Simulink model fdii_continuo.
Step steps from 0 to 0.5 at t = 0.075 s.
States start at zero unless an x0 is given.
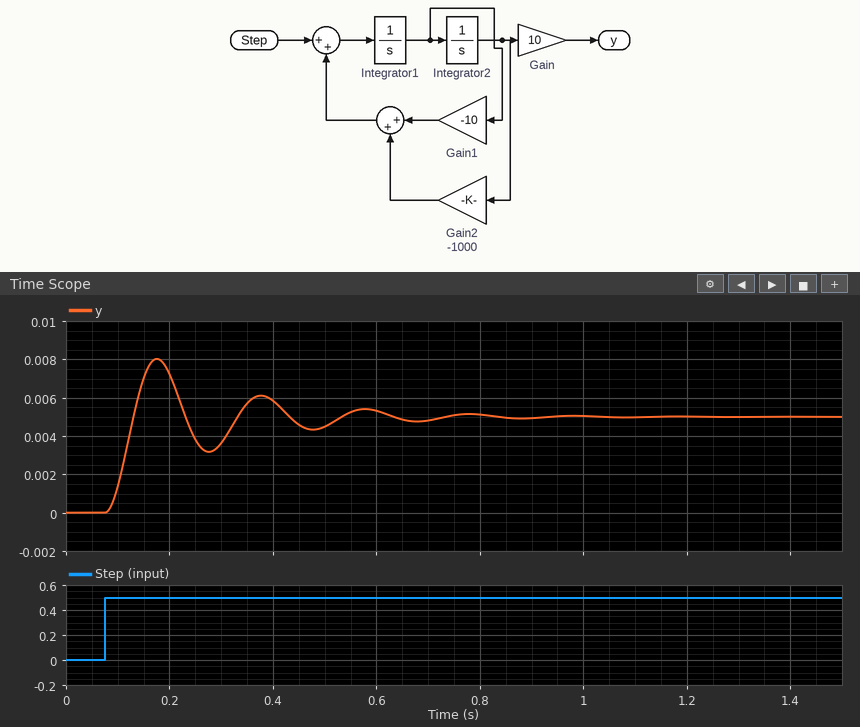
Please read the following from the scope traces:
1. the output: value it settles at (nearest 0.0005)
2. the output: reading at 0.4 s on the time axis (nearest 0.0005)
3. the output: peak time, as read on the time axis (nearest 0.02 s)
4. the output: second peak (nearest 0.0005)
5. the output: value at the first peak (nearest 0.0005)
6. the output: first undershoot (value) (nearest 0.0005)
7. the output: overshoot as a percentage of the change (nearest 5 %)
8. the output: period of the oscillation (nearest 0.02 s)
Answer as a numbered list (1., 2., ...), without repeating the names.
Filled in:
1. 0.0050
2. 0.0060
3. 0.18 s
4. 0.0060
5. 0.0080
6. 0.0030
7. 60 %
8. 0.20 s
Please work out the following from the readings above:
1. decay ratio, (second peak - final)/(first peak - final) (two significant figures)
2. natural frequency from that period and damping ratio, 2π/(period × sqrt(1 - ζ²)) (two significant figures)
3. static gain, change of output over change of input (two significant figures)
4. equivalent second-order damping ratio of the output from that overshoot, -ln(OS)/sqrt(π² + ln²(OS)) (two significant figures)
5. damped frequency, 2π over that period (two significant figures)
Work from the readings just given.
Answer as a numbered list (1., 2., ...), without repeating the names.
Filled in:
1. 0.33
2. 32 rad/s
3. 0.010
4. 0.16
5. 31 rad/s
